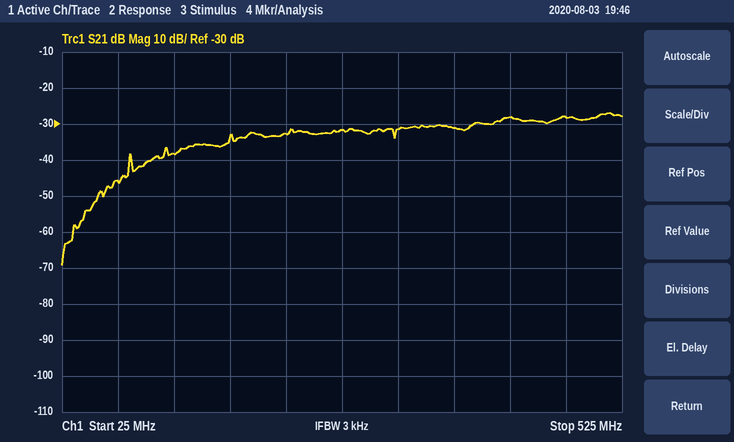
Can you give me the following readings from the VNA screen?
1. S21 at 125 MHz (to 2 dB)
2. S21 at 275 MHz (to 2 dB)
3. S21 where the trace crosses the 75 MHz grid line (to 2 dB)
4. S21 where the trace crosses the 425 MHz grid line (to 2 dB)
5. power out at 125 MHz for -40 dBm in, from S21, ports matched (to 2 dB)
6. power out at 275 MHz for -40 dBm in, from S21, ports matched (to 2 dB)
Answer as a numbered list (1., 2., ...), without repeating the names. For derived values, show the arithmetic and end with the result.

1. -38 dB
2. -32 dB
3. -46 dB
4. -28 dB
5. -40 dBm + (-38 dB) = -78 dBm
6. -40 dBm + (-32 dB) = -72 dBm
